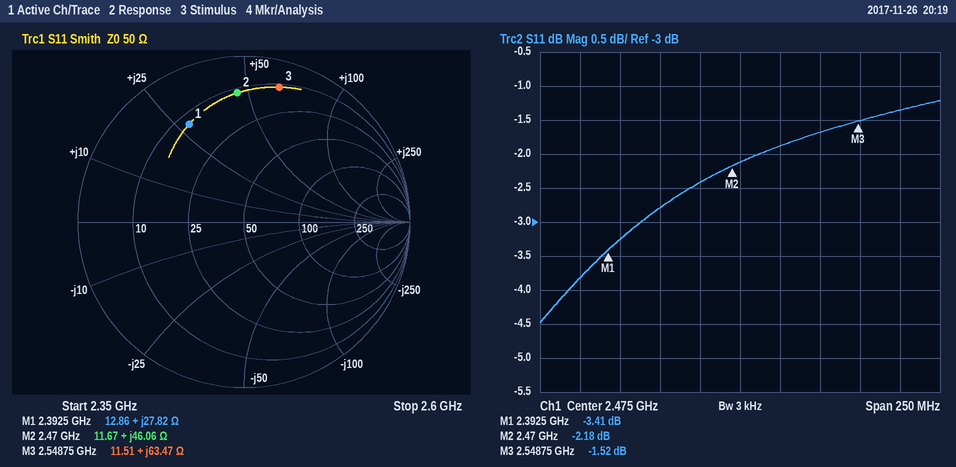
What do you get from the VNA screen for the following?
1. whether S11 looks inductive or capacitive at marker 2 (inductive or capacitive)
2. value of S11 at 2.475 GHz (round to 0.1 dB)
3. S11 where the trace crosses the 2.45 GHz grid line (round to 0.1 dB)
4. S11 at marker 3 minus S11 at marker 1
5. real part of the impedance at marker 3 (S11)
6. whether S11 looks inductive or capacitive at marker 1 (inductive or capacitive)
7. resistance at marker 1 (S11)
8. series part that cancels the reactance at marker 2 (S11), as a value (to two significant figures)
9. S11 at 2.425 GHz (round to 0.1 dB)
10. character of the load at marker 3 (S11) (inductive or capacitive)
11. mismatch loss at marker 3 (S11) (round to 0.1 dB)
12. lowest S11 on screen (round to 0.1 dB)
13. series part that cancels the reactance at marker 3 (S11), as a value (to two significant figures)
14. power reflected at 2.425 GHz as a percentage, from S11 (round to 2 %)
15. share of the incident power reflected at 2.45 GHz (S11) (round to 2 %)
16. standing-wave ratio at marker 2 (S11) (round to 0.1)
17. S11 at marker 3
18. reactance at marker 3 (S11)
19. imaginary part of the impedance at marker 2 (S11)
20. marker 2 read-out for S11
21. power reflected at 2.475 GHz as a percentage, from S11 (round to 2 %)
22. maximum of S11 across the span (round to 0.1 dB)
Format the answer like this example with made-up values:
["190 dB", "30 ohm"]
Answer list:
["inductive", "-2.1 dB", "-2.4 dB", "1.89 dB", "11.51 Ω", "inductive", "12.86 Ω", "1.4 pF", "-2.8 dB", "inductive", "5.3 dB", "-4.5 dB", "980 fF", "52 %", "58 %", "8.0", "-1.52 dB", "+63.47 Ω", "+46.06 Ω", "-2.18 dB", "62 %", "-1.2 dB"]
